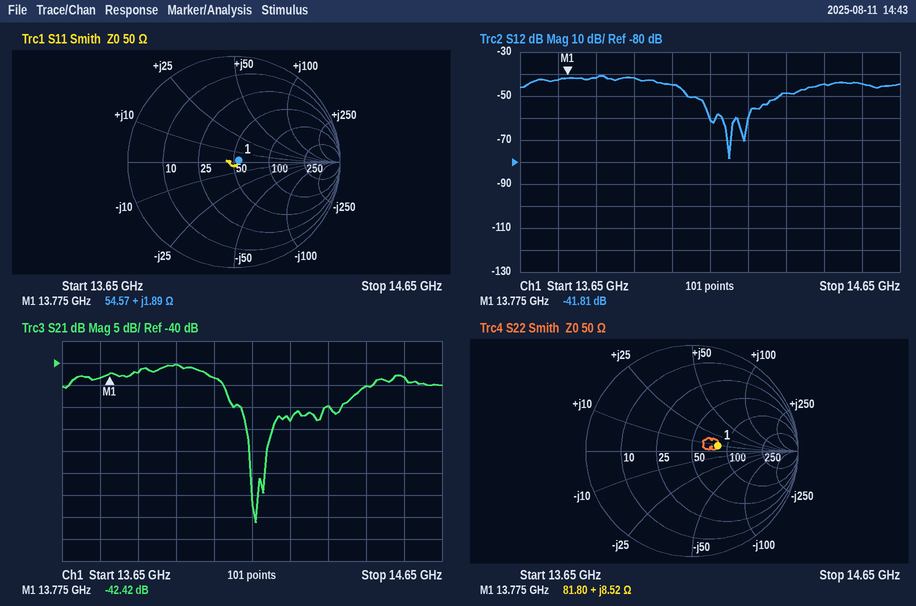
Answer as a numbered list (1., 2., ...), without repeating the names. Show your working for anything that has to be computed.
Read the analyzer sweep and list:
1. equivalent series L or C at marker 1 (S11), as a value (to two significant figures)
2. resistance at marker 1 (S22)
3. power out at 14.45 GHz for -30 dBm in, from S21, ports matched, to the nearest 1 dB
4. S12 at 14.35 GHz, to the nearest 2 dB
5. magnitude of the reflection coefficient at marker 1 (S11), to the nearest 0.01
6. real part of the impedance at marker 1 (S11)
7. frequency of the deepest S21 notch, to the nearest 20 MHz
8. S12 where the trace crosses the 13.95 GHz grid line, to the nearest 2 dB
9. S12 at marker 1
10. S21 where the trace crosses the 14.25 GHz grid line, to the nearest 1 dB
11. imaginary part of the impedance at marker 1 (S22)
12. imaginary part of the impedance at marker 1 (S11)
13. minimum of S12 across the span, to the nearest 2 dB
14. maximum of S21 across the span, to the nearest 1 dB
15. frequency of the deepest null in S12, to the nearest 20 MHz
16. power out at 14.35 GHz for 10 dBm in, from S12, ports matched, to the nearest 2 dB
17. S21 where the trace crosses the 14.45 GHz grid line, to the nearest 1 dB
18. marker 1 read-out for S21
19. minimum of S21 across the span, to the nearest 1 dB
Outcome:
1. L = 1.89 Ω/(2π × 13.775 GHz) ≈ 22 pH
2. 81.80 Ω
3. -30 dBm + (-45 dB) = -75 dBm
4. -48 dB
5. 0.05
6. 54.57 Ω
7. 14.16 GHz
8. -42 dB
9. -41.81 dB
10. -53 dB
11. +8.52 Ω
12. +1.89 Ω
13. -78 dB
14. -40 dB
15. 14.20 GHz
16. 10 dBm + (-48 dB) = -38 dBm
17. -45 dB
18. -42.42 dB
19. -76 dB
